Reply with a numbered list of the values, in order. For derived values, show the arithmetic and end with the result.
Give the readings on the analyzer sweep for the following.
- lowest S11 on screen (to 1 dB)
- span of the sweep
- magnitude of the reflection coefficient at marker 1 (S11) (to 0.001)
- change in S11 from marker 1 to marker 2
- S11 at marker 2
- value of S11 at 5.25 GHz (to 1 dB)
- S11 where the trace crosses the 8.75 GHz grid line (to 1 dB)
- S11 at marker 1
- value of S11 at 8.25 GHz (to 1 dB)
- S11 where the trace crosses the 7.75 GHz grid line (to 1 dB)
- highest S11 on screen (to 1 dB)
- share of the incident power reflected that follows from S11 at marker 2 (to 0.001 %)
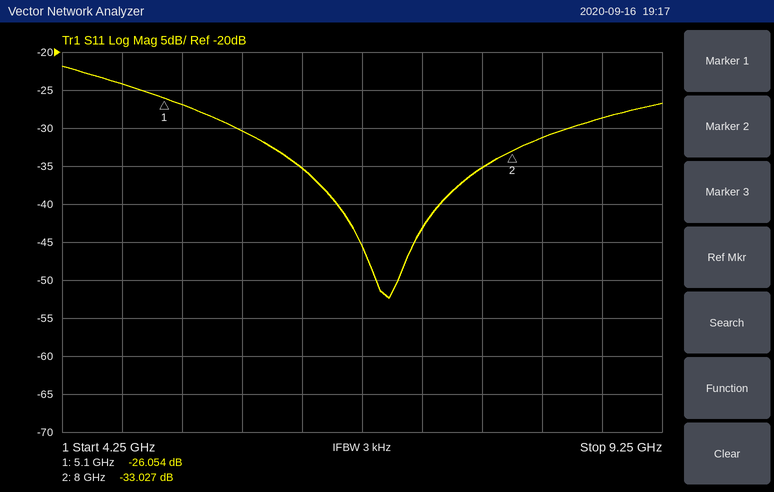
1. -52 dB
2. 5 GHz
3. 10^(-26.054/20) ≈ 0.050
4. -33.027 − (-26.054) = -6.973 dB
5. -33.027 dB
6. -27 dB
7. -29 dB
8. -26.054 dB
9. -31 dB
10. -35 dB
11. -22 dB
12. 10^(-33.027/10) ≈ 0.050 %
